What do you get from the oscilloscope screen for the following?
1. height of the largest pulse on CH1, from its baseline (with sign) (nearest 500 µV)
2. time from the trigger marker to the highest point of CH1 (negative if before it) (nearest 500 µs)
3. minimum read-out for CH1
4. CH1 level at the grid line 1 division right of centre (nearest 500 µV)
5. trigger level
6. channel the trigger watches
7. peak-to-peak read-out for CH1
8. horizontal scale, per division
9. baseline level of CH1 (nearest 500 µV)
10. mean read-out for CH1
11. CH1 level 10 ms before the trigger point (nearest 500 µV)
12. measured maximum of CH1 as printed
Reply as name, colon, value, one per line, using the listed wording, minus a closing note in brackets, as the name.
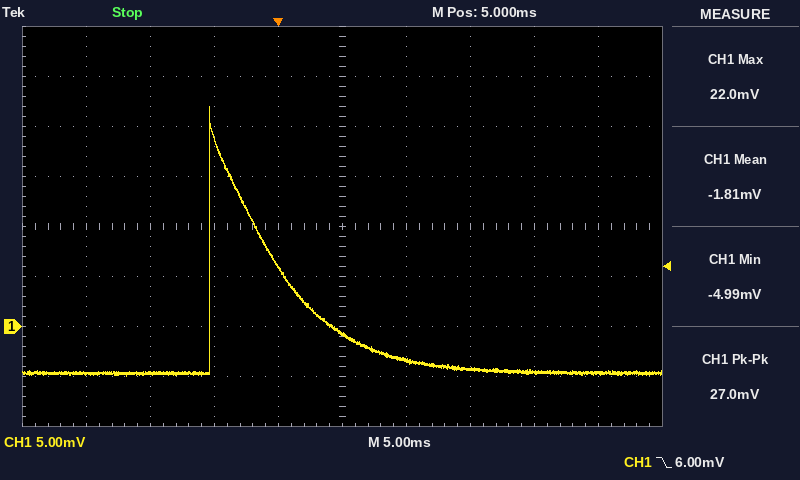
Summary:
height of the largest pulse on CH1, from its baseline (with sign): +26.5 mV
time from the trigger marker to the highest point of CH1 (negative if before it): -5.5 ms
minimum read-out for CH1: -4.99 mV
CH1 level at the grid line 1 division right of centre: -3.5 mV
trigger level: 6.00 mV
channel the trigger watches: CH1
peak-to-peak read-out for CH1: 27.0 mV
horizontal scale, per division: 5 ms
baseline level of CH1: -4.5 mV
mean read-out for CH1: -1.81 mV
CH1 level 10 ms before the trigger point: -4.5 mV
measured maximum of CH1 as printed: 22.0 mV
